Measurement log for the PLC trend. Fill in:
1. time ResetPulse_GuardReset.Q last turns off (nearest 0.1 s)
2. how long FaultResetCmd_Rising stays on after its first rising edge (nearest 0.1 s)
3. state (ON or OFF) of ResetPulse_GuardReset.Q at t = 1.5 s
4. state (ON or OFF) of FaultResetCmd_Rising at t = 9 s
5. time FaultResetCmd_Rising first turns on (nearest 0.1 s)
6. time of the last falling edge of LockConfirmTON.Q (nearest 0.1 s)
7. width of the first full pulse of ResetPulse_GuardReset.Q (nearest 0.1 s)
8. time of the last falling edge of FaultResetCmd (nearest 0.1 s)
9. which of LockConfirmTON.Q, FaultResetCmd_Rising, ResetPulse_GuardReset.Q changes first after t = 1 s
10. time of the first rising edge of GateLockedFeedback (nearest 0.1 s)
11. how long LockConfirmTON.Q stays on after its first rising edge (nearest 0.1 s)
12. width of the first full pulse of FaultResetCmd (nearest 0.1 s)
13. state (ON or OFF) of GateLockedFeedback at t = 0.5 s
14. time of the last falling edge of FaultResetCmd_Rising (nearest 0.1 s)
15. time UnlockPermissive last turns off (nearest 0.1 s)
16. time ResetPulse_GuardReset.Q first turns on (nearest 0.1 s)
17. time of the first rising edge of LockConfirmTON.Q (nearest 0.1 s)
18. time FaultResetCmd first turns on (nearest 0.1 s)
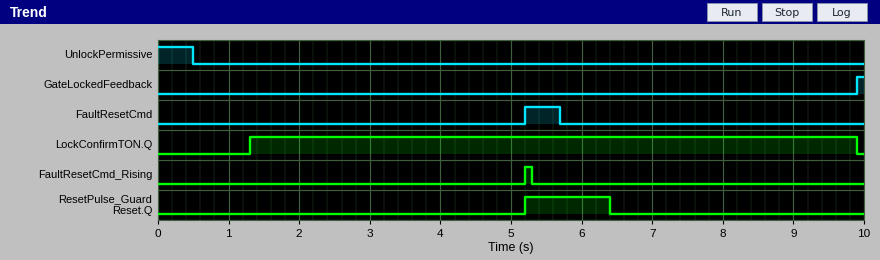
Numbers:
6.4 s
0.1 s
OFF
OFF
5.2 s
9.9 s
1.2 s
5.7 s
LockConfirmTON.Q
9.9 s
8.6 s
0.5 s
OFF
5.3 s
0.5 s
5.2 s
1.3 s
5.2 s
